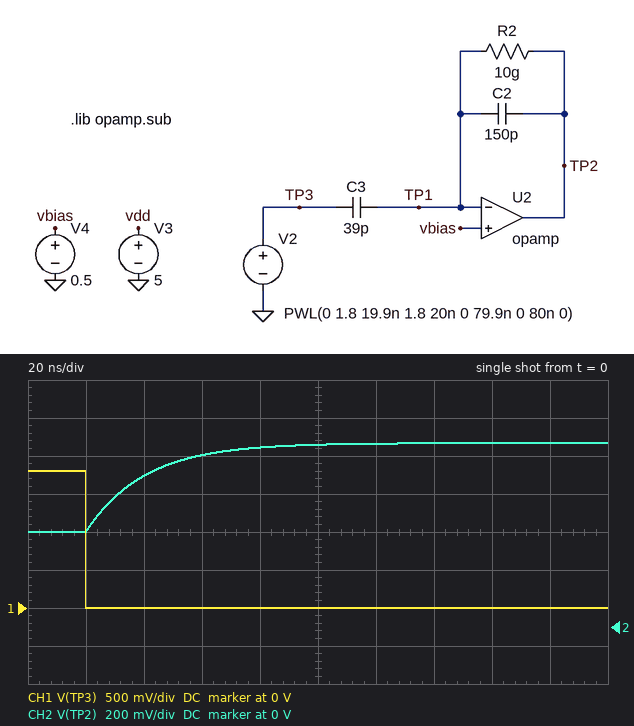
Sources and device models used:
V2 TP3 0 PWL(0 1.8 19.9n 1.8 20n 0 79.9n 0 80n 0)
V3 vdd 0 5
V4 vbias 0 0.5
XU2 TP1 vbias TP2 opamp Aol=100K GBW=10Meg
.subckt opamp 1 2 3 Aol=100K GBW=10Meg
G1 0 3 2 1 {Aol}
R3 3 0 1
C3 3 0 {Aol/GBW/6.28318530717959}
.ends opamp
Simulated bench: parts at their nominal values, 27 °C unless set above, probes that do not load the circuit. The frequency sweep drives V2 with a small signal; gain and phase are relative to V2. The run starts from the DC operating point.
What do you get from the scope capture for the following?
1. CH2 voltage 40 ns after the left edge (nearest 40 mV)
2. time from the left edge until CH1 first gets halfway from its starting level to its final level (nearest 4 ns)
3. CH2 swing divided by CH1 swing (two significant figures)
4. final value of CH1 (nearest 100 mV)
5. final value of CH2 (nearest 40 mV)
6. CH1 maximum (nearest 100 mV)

800 mV
20 ns
0.26
0 V
960 mV
1.8 V
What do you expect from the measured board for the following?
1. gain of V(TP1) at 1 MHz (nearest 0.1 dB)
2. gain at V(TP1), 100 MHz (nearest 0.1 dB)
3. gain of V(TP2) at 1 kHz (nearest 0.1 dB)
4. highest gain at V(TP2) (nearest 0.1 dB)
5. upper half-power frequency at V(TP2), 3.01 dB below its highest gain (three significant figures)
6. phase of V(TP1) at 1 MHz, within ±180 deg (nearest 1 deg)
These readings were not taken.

-31.8 dB
-13.7 dB
-11.7 dB
-11.7 dB
7.94 MHz
83 deg
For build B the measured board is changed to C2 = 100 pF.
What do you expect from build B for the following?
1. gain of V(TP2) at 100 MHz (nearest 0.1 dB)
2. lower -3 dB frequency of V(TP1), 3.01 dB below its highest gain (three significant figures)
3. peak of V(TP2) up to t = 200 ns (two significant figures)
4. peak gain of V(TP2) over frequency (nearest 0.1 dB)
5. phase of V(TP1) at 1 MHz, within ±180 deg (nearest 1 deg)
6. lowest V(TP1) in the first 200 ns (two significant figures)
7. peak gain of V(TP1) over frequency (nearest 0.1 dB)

-31.1 dB
7.19 MHz
1.2 V
-8.2 dB
82 deg
-3.9 mV
-11.0 dB
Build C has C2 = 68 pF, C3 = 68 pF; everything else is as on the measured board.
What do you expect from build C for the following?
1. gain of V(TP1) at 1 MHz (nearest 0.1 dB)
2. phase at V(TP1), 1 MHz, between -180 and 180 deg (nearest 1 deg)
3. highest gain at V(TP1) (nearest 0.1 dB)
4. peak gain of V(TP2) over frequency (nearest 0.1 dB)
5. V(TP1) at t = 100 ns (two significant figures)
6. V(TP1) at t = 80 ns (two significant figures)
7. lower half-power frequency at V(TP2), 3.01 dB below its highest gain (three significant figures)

-20.2 dB
79 deg
-6.0 dB
0 dB
430 mV
360 mV
234 mHz
